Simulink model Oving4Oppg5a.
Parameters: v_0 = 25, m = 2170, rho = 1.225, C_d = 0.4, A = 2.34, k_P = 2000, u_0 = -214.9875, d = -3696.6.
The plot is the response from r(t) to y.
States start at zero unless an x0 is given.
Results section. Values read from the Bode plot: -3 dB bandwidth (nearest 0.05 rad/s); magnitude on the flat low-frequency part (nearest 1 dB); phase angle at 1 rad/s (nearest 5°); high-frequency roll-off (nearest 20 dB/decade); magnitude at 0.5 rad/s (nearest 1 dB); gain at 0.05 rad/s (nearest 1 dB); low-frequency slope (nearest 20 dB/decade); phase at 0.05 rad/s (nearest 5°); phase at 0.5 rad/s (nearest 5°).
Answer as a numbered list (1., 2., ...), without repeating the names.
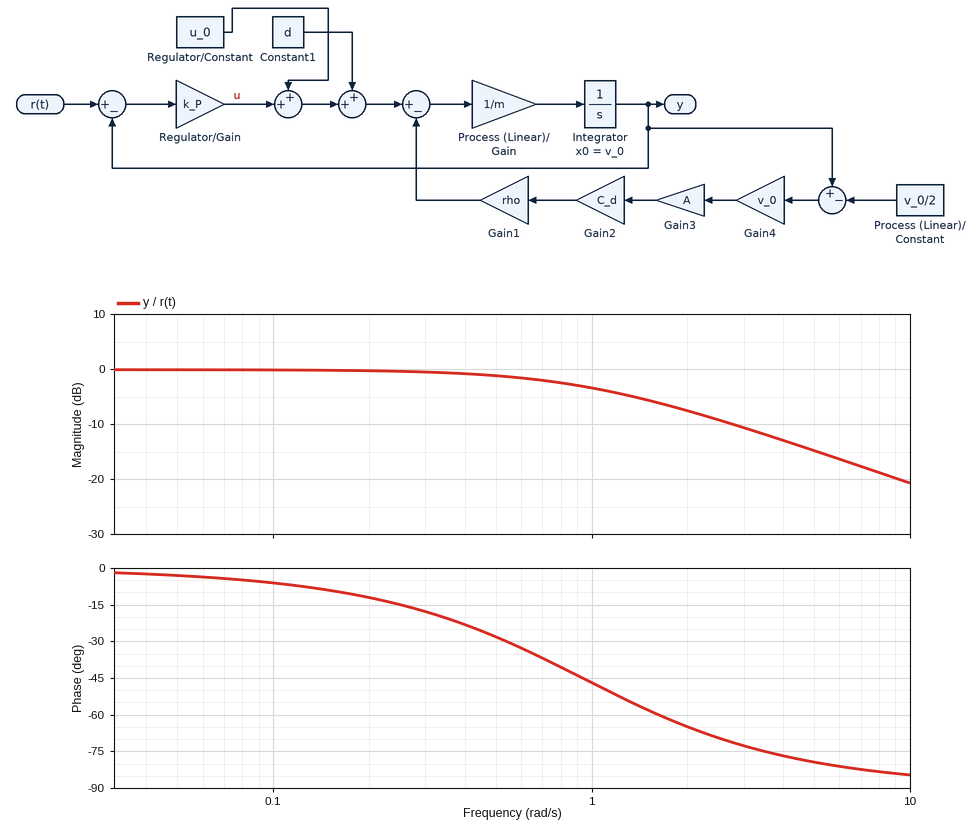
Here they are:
1. 0.95 rad/s
2. 0 dB
3. -45°
4. -20 dB/decade
5. -1 dB
6. 0 dB
7. 0 dB/decade
8. -5°
9. -30°
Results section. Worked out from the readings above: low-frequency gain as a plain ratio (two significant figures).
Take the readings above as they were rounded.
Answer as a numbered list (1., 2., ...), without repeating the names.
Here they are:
1. 1.0
